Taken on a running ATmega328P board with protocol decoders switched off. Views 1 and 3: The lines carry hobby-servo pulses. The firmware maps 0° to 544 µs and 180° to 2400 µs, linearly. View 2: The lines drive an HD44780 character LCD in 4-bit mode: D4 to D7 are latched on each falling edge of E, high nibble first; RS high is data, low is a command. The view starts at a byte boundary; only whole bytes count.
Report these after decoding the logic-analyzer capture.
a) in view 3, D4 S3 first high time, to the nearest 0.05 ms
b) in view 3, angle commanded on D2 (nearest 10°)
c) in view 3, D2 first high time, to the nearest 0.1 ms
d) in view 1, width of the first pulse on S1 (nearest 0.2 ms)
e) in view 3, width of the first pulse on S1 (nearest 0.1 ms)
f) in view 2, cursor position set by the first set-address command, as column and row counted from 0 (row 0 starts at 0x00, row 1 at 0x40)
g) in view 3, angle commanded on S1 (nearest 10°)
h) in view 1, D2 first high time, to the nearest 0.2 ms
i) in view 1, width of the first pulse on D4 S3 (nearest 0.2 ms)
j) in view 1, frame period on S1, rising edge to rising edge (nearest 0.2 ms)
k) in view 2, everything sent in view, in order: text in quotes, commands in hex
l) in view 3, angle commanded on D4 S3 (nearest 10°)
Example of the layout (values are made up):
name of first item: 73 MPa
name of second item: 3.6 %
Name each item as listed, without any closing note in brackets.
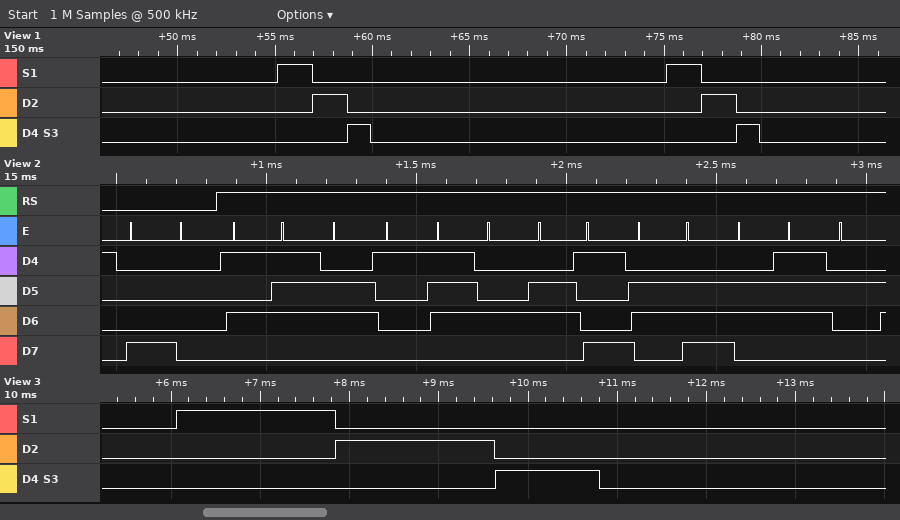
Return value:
in view 3, D4 S3 first high time, to the nearest 0.05 ms: 1.15 ms
in view 3, angle commanded on D2: 120°
in view 3, D2 first high time, to the nearest 0.1 ms: 1.8 ms
in view 1, width of the first pulse on S1: 1.8 ms
in view 3, width of the first pulse on S1: 1.8 ms
in view 2, cursor position set by the first set-address command, as column and row counted from 0: column 0, row 0
in view 3, angle commanded on S1: 120°
in view 1, D2 first high time, to the nearest 0.2 ms: 1.8 ms
in view 1, width of the first pulse on D4 S3: 1.2 ms
in view 1, frame period on S1, rising edge to rising edge: 20.0 ms
in view 2, everything sent in view, in order: text in quotes, commands in hex: 0x80 "Wating"
in view 3, angle commanded on D4 S3: 60°
